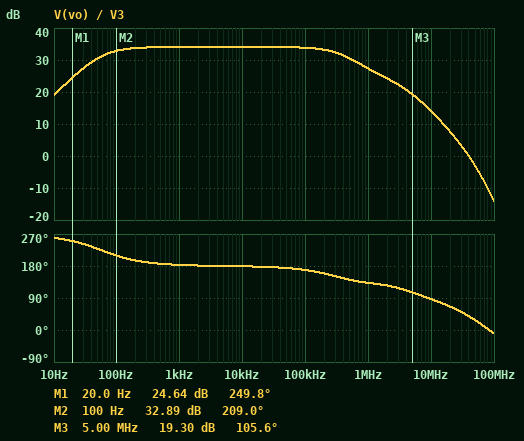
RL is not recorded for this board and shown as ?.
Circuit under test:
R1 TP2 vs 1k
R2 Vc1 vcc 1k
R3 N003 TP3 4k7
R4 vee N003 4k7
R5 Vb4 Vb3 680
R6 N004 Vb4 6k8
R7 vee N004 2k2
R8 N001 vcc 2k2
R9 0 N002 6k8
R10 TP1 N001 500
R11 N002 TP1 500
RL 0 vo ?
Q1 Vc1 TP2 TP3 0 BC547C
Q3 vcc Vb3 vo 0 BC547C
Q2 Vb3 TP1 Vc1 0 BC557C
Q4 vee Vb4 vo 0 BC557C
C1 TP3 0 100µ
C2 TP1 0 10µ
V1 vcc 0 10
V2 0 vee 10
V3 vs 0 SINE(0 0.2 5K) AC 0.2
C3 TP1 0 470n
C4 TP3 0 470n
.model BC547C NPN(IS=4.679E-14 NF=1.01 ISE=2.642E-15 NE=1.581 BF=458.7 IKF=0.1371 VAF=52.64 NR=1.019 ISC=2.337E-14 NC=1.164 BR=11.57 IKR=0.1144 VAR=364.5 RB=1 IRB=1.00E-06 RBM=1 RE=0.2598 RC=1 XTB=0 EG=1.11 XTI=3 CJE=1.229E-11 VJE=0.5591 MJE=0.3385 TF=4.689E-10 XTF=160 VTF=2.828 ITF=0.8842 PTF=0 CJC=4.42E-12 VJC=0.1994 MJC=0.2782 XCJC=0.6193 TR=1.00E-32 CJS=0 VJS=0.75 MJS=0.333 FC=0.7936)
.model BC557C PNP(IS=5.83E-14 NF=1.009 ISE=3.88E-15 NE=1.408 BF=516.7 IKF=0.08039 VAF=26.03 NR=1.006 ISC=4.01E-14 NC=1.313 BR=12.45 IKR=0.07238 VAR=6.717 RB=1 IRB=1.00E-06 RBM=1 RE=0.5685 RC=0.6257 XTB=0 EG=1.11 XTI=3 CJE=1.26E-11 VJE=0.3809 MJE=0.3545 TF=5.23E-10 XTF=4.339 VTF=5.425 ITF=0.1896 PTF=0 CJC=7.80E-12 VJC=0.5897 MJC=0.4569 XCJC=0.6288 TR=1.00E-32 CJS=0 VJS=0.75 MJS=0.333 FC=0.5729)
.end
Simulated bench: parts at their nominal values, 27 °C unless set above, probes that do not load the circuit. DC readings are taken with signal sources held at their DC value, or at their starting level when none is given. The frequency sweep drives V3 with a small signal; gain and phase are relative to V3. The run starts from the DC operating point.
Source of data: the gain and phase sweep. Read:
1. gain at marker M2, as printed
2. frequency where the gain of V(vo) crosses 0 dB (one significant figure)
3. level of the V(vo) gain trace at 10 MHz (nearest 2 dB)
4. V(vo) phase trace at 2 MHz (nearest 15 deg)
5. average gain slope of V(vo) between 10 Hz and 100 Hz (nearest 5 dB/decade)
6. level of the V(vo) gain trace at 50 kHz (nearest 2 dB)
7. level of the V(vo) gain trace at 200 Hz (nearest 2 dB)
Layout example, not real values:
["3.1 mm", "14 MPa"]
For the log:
["32.89 dB", "40 MHz", "14 dB", "120 deg", "15 dB/decade", "34 dB", "34 dB"]
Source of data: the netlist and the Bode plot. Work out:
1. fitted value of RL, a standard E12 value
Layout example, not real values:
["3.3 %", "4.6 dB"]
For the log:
["560 Ω"]
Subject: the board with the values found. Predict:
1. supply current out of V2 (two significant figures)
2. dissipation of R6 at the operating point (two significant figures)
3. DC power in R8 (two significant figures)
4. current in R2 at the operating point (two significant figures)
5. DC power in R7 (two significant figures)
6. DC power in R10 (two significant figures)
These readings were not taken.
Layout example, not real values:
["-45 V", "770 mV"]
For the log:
["2.1 mA", "8.0 mW", "2.2 mW", "2.1 mA", "2.6 mW", "500 µW"]
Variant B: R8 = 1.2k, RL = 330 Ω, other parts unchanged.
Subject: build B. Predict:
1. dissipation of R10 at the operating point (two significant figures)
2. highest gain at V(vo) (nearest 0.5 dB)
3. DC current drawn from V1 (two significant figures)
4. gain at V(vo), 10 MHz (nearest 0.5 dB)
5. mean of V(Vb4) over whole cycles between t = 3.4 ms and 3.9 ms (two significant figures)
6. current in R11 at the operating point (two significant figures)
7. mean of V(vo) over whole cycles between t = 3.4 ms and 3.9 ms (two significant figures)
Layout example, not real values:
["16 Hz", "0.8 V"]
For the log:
["620 µW", "48.5 dB", "2.4 mA", "23.5 dB", "-2.8 V", "1.1 mA", "-2.4 V"]
